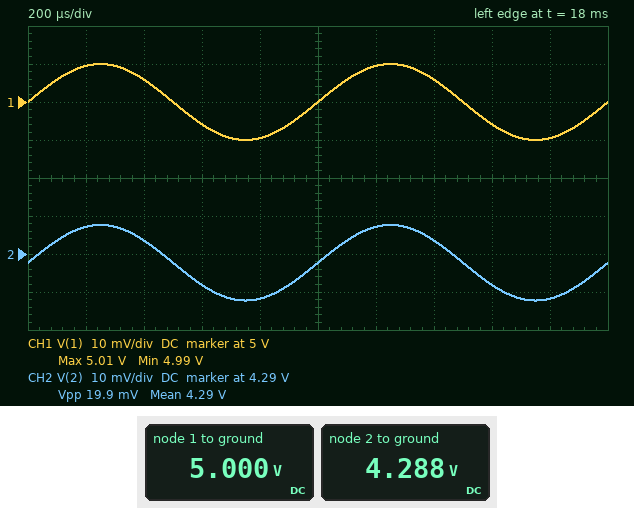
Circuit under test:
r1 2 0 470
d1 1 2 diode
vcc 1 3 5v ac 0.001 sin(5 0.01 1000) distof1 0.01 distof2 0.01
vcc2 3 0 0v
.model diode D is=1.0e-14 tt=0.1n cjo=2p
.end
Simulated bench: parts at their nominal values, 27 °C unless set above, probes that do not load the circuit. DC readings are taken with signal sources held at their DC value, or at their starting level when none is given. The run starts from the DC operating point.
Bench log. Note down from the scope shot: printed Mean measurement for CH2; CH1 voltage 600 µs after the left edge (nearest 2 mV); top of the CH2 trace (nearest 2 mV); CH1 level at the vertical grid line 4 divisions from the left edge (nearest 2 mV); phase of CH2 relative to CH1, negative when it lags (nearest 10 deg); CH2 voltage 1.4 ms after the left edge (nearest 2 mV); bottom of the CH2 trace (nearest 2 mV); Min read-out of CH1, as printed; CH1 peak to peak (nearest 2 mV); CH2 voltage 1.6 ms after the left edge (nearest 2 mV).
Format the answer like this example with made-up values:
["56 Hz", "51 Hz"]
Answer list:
["4.29 V", "4.994 V", "4.298 V", "4.990 V", "0 deg", "4.294 V", "4.278 V", "4.99 V", "20 mV", "4.282 V"]
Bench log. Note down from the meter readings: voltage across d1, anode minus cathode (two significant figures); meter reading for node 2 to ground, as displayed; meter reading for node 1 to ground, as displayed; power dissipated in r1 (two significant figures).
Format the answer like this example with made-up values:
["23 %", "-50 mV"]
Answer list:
["710 mV", "4.288 V", "5.000 V", "39 mW"]
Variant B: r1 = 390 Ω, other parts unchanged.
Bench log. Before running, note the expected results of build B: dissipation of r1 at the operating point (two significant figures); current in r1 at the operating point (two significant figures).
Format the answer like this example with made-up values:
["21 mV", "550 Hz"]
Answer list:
["47 mW", "11 mA"]
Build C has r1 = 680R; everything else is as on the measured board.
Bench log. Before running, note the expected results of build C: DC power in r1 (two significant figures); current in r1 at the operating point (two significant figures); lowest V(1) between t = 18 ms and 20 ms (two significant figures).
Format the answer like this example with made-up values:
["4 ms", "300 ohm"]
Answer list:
["27 mW", "6.3 mA", "5.0 V"]
